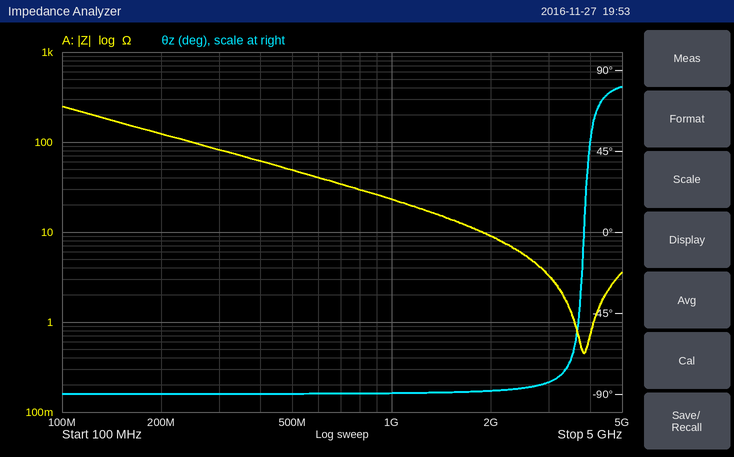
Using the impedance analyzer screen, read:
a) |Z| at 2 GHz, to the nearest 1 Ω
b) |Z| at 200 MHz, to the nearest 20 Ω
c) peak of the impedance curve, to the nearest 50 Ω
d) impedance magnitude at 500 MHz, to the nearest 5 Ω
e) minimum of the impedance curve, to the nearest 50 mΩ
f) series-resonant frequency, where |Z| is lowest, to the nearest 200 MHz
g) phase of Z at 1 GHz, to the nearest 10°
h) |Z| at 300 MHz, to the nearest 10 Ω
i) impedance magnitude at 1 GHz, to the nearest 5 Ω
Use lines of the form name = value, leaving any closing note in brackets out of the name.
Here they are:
|Z| at 2 GHz, to the nearest 1 Ω = 9 Ω
|Z| at 200 MHz, to the nearest 20 Ω = 120 Ω
peak of the impedance curve, to the nearest 50 Ω = 250 Ω
impedance magnitude at 500 MHz, to the nearest 5 Ω = 50 Ω
minimum of the impedance curve, to the nearest 50 mΩ = 450 mΩ
series-resonant frequency, where |Z| is lowest, to the nearest 200 MHz = 3.8 GHz
phase of Z at 1 GHz, to the nearest 10° = -90°
|Z| at 300 MHz, to the nearest 10 Ω = 80 Ω
impedance magnitude at 1 GHz, to the nearest 5 Ω = 25 Ω
